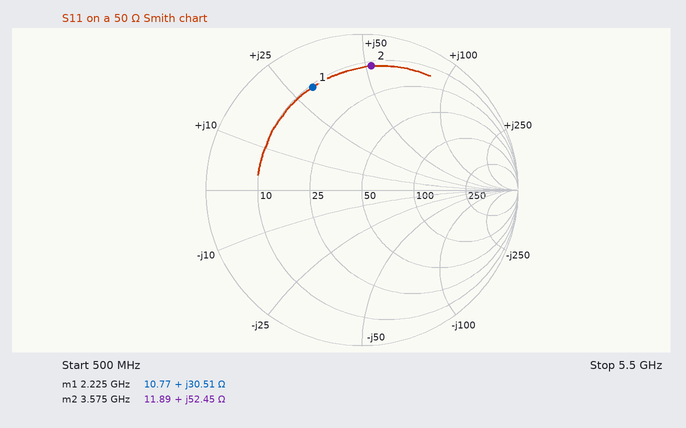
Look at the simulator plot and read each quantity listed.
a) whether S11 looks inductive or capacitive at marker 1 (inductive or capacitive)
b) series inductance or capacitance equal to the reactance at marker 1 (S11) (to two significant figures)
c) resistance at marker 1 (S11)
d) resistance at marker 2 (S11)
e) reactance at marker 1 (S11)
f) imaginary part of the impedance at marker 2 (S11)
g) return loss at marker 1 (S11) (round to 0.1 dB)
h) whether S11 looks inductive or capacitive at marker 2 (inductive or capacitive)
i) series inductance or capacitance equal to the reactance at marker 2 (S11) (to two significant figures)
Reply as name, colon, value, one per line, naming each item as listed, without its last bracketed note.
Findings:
whether S11 looks inductive or capacitive at marker 1: inductive
series inductance or capacitance equal to the reactance at marker 1 (S11): 2.2 nH
resistance at marker 1: 10.77 Ω
resistance at marker 2: 11.89 Ω
reactance at marker 1: +30.51 Ω
imaginary part of the impedance at marker 2: +52.45 Ω
return loss at marker 1 (S11): 2.7 dB
whether S11 looks inductive or capacitive at marker 2: inductive
series inductance or capacitance equal to the reactance at marker 2 (S11): 2.3 nH
